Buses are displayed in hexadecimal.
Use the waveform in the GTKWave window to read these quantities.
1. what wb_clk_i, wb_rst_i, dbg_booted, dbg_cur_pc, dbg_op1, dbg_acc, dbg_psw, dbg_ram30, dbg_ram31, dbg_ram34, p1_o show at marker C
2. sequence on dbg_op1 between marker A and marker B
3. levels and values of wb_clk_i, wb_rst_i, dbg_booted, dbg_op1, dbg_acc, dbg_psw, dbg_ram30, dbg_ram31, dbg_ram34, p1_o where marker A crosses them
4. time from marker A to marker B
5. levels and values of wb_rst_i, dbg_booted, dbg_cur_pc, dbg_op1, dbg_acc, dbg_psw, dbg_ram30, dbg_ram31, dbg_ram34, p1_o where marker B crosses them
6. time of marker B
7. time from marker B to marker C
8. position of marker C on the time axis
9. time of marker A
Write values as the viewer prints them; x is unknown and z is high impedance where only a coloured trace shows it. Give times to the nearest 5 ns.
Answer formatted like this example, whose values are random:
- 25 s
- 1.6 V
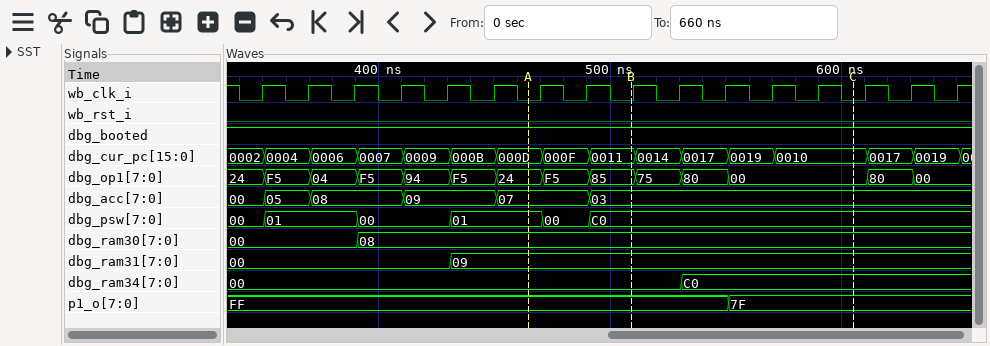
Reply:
- wb_clk_i=0, wb_rst_i=0, dbg_booted=1, dbg_cur_pc=0010, dbg_op1=00, dbg_acc=03, dbg_psw=C0, dbg_ram30=08, dbg_ram31=09, dbg_ram34=C0, p1_o=7F
- 24, F5, 85
- wb_clk_i=0, wb_rst_i=0, dbg_booted=1, dbg_op1=24, dbg_acc=07, dbg_psw=01, dbg_ram30=08, dbg_ram31=09, dbg_ram34=00, p1_o=FF
- 45 ns
- wb_rst_i=0, dbg_booted=1, dbg_cur_pc=0011, dbg_op1=85, dbg_acc=03, dbg_psw=C0, dbg_ram30=08, dbg_ram31=09, dbg_ram34=00, p1_o=FF
- 510 ns
- 95 ns
- 605 ns
- 465 ns
